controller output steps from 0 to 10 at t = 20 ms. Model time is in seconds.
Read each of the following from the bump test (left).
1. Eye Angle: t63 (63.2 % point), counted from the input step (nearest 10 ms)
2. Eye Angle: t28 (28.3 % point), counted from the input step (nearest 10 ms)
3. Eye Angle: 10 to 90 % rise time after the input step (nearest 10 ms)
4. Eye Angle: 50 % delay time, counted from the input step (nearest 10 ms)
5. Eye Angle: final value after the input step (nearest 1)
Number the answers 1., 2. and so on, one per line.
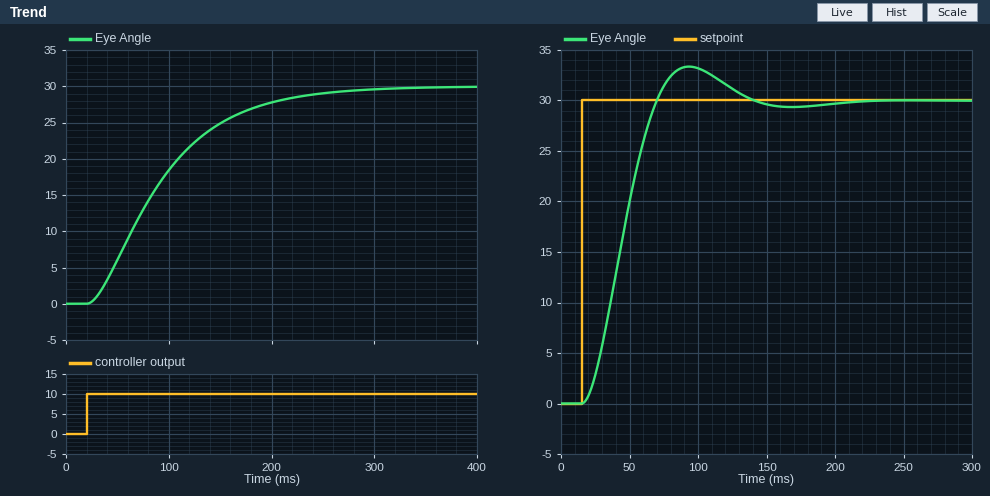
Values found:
1. 80 ms
2. 40 ms
3. 140 ms
4. 60 ms
5. 30
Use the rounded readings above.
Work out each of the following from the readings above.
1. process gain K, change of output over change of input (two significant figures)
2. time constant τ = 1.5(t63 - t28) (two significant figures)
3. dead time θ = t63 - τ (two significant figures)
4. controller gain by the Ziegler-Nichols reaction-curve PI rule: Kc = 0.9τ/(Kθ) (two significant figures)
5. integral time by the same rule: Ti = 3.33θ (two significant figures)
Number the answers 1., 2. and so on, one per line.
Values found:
1. 3.0
2. 60 ms
3. 20 ms
4. 0.90
5. 67 ms
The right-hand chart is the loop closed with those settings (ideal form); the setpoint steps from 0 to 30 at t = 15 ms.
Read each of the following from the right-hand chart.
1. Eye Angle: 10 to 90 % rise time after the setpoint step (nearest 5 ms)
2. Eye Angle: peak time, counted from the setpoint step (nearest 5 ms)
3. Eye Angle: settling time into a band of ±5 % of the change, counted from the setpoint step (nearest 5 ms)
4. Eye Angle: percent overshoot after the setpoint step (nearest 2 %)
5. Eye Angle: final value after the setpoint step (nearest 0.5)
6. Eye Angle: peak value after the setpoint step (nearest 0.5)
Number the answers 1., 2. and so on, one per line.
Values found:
1. 35 ms
2. 80 ms
3. 105 ms
4. 12 %
5. 30.0
6. 33.5
